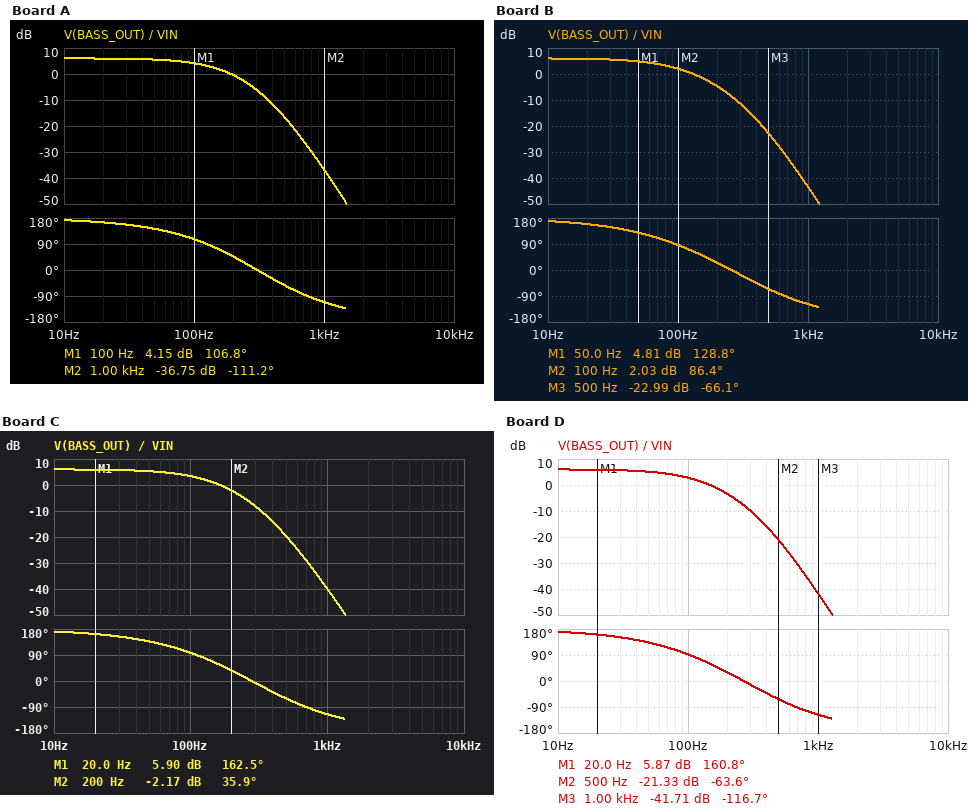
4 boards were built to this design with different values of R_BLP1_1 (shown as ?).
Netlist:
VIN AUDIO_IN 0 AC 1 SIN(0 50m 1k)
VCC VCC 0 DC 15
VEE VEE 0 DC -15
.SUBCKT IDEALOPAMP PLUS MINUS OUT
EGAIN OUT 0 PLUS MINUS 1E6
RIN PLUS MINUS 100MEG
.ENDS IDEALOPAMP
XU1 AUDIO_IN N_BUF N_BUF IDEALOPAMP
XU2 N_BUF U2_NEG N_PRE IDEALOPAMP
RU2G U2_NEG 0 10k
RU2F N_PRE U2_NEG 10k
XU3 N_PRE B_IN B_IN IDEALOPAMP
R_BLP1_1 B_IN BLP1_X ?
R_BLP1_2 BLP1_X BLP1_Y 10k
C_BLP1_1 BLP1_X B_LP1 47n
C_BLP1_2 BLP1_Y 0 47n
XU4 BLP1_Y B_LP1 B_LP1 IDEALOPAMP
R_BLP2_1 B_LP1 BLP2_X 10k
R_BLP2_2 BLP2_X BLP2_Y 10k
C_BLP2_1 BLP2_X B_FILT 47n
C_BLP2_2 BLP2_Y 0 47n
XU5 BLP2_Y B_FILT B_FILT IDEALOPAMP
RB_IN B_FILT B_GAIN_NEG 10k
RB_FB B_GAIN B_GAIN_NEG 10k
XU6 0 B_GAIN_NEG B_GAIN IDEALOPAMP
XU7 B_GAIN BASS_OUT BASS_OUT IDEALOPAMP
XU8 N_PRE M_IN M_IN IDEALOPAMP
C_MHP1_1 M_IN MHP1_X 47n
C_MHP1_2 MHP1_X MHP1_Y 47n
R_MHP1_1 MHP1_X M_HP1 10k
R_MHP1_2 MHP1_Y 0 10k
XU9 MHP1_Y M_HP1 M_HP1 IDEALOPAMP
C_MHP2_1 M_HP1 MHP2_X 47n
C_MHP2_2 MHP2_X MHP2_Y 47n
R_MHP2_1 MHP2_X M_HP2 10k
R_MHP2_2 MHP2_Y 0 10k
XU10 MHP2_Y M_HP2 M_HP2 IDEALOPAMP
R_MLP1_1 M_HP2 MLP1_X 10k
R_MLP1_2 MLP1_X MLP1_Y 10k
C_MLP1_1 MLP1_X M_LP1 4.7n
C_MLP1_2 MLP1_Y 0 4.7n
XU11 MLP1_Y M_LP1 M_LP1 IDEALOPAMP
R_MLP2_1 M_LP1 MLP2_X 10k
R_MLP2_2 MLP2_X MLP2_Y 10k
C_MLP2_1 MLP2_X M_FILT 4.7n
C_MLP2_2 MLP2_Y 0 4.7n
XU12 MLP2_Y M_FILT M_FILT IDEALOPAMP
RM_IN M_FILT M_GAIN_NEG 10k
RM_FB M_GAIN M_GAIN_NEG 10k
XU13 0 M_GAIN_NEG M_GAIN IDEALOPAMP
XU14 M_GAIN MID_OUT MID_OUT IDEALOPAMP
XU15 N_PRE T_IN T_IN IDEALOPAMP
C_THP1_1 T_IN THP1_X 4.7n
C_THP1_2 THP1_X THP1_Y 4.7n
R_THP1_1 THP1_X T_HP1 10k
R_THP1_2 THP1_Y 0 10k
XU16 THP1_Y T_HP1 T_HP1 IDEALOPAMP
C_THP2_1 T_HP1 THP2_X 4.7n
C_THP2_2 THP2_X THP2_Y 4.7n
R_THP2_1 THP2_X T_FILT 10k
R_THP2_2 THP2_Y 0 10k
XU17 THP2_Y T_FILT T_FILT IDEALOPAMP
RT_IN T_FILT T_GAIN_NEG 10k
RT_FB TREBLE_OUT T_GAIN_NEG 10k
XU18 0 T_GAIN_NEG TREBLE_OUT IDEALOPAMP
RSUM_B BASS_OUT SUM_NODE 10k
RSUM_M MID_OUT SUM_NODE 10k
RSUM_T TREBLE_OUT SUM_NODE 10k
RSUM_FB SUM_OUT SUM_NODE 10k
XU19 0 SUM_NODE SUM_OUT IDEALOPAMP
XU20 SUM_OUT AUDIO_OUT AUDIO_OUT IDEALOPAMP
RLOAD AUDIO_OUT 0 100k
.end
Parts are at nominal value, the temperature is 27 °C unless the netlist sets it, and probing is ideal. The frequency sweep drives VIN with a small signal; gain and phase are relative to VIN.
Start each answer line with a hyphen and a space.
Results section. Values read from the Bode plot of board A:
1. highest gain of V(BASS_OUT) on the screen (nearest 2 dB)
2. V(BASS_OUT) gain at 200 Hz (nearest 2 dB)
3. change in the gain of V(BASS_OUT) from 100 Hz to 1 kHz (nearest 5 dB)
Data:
- 6 dB
- 0 dB
- -40 dB
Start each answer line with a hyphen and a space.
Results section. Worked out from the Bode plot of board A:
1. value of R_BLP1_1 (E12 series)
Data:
- 15 kΩ
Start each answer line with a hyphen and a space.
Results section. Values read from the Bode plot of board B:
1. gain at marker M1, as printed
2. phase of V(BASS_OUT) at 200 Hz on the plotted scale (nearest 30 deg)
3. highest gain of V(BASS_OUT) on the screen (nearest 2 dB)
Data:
- 4.81 dB
- 30 deg
- 6 dB
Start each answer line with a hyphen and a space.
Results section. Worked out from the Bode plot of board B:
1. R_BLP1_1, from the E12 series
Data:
- 33 kΩ
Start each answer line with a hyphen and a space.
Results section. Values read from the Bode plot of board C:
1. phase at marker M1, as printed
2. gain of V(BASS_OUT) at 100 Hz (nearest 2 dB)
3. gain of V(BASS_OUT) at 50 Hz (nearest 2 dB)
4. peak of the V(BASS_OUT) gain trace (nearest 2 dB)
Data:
- 162.5 deg
- 4 dB
- 6 dB
- 6 dB
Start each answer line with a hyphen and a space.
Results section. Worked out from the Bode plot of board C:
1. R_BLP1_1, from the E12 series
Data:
- 22 kΩ
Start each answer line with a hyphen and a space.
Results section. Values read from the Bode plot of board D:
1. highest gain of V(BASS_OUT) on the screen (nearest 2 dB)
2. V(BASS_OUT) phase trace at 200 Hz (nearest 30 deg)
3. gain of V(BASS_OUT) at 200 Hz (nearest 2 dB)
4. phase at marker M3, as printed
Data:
- 6 dB
- 30 deg
- -4 dB
- -116.7 deg
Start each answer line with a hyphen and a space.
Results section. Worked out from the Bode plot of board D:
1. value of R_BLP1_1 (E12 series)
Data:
- 27 kΩ
